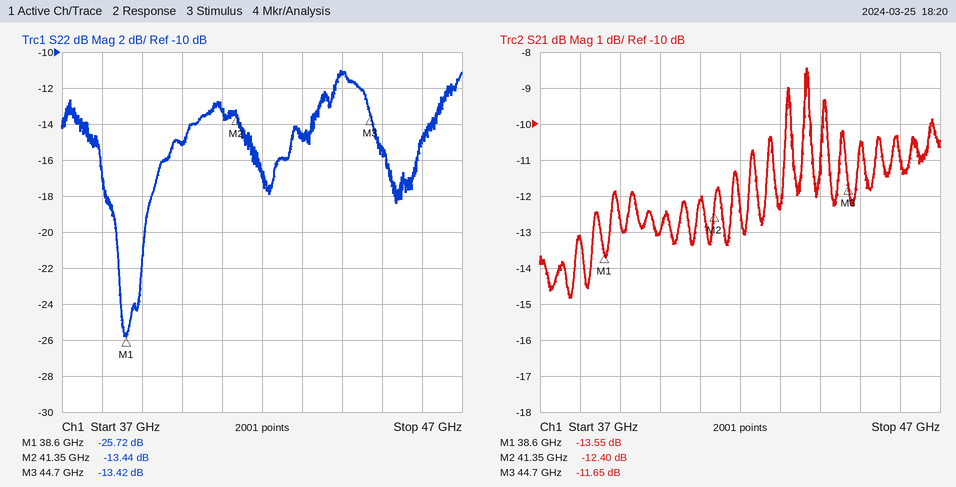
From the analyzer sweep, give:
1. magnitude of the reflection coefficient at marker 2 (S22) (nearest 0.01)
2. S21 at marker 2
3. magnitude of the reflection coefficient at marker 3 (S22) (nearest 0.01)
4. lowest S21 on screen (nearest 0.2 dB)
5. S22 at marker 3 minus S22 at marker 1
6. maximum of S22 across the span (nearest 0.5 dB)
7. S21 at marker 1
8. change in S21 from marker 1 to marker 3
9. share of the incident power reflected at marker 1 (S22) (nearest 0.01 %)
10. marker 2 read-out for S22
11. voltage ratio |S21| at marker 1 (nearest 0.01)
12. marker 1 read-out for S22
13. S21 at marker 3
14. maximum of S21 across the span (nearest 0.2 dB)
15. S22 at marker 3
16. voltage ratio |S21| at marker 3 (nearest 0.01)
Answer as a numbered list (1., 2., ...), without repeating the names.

1. 0.21
2. -12.40 dB
3. 0.21
4. -14.8 dB
5. 12.30 dB
6. -11.0 dB
7. -13.55 dB
8. 1.90 dB
9. 0.27 %
10. -13.44 dB
11. 0.21
12. -25.72 dB
13. -11.65 dB
14. -8.4 dB
15. -13.42 dB
16. 0.26
